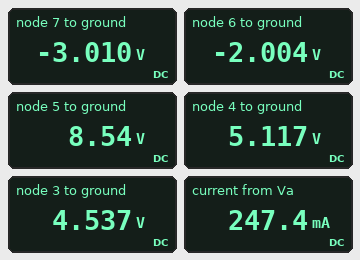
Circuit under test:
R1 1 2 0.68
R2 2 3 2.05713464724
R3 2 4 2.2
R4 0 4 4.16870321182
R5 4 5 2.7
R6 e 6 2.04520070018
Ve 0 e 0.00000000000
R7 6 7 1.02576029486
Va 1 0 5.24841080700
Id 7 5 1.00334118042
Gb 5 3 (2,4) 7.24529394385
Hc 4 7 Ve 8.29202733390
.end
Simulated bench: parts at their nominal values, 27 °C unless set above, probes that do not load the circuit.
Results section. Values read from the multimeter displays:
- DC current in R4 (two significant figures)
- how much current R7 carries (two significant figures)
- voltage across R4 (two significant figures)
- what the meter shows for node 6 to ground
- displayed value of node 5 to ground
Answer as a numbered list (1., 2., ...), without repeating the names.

1. 1.2 A
2. 980 mA
3. 5.1 V
4. -2.004 V
5. 8.54 V
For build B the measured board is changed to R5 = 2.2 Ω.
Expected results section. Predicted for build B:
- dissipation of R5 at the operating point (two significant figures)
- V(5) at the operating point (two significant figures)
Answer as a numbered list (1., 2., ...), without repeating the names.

1. 3.5 W
2. 7.9 V
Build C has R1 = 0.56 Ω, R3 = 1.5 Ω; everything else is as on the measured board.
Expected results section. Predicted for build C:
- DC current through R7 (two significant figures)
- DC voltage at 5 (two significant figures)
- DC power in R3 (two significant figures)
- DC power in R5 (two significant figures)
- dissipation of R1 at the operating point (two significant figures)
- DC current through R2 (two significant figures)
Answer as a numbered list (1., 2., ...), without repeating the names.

1. 990 mA
2. 8.6 V
3. 950 µW
4. 4.4 W
5. 35 mW
6. 270 mA
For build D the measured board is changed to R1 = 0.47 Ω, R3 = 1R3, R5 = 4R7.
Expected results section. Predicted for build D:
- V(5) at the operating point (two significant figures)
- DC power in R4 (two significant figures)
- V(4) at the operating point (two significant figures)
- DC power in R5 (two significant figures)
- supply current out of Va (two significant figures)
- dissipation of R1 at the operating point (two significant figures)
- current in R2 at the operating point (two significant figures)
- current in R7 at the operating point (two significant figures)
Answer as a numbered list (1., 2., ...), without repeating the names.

1. 11 V
2. 6.4 W
3. 5.2 V
4. 7.7 W
5. 250 mA
6. 29 mW
7. 280 mA
8. 990 mA
